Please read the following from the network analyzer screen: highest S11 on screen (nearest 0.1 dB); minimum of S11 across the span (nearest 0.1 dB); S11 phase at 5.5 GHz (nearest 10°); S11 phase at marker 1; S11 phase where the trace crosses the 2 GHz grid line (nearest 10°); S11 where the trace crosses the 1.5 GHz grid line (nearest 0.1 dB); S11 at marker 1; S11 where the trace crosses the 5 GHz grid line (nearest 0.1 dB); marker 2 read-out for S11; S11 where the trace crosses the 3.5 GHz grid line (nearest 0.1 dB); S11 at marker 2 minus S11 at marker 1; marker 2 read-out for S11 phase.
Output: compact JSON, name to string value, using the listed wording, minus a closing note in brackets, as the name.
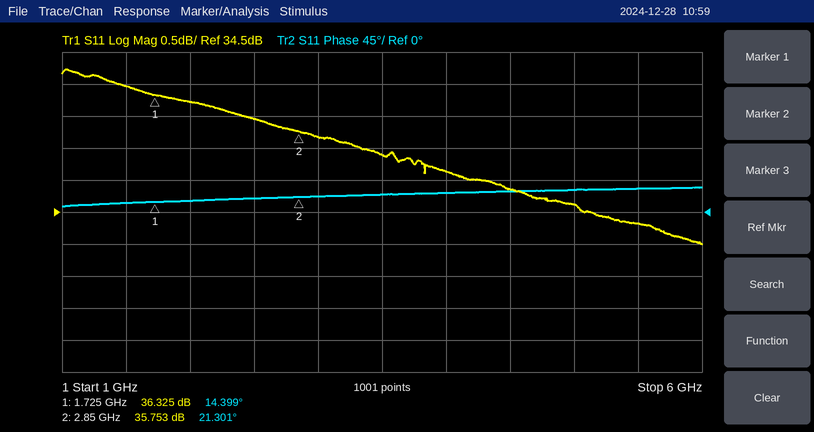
{"highest S11 on screen": "36.7 dB", "minimum of S11 across the span": "34.0 dB", "S11 phase at 5.5 GHz": "30°", "S11 phase at marker 1": "14.399°", "S11 phase where the trace crosses the 2 GHz grid line": "20°", "S11 where the trace crosses the 1.5 GHz grid line": "36.5 dB", "S11 at marker 1": "36.325 dB", "S11 where the trace crosses the 5 GHz grid line": "34.6 dB", "marker 2 read-out for S11": "35.753 dB", "S11 where the trace crosses the 3.5 GHz grid line": "35.4 dB", "S11 at marker 2 minus S11 at marker 1": "-0.572 dB", "marker 2 read-out for S11 phase": "21.301°"}
